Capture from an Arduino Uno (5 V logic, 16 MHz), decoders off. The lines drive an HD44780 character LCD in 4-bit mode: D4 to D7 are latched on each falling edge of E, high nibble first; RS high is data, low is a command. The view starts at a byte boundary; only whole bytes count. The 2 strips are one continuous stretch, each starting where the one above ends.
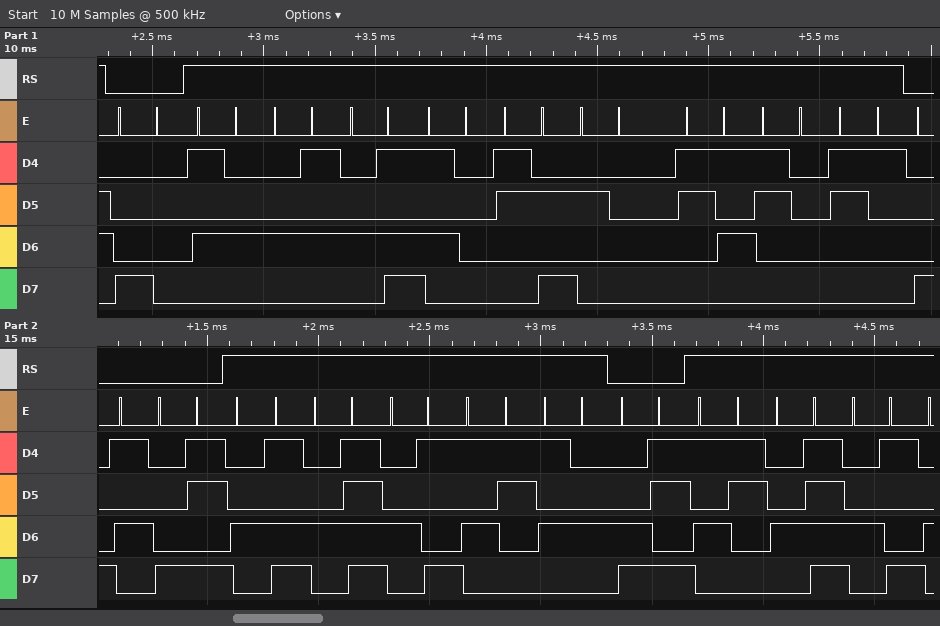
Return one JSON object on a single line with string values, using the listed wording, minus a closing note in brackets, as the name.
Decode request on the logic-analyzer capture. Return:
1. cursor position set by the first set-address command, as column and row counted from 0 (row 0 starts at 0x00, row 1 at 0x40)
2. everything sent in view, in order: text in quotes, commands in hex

{"cursor position set by the first set-address command, as column and row counted from 0": "column 0, row 0", "everything sent in view, in order: text in quotes, commands in hex": "0x80 \"TEMP: 501\" 0x85 0x8B \"MOIST\" 0xCB \"SOI\""}
